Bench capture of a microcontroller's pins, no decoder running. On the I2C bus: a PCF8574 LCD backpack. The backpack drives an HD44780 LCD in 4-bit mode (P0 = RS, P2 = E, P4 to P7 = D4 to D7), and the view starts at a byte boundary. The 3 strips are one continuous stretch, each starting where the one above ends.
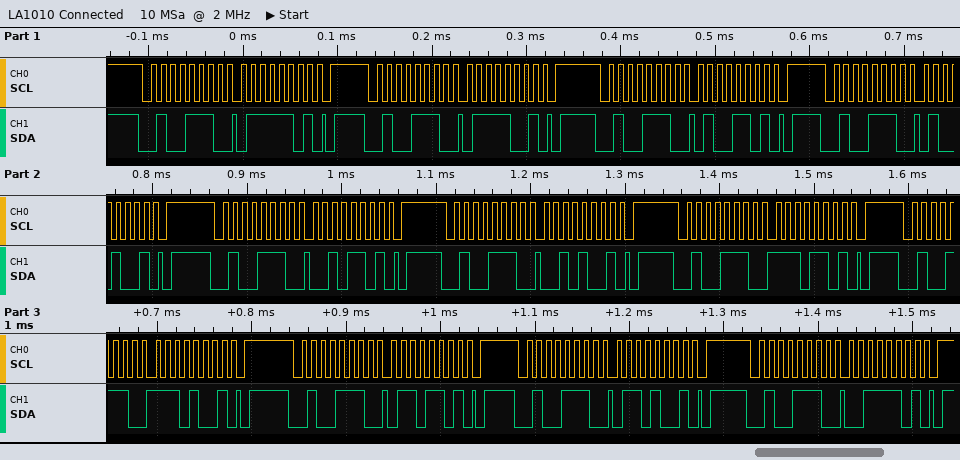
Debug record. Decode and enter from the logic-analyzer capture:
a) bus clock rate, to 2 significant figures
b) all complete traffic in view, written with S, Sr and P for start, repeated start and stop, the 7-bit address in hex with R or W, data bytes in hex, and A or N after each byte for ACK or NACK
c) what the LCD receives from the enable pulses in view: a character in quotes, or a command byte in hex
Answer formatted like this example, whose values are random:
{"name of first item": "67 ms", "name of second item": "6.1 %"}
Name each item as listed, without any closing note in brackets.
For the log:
{"bus clock rate, to 2 significant figures": "100 kHz", "all complete traffic in view, written with S, Sr and P for start, repeated start and stop, the 7-bit address in hex with R or W, data bytes in hex, and A or N after each byte for ACK or NACK": "S 27W A 7D A P S 27W A 79 A P S 27W A 4D A P S 27W A 49 A P S 27W A 2D A P S 27W A 29 A P S 27W A ED A P S 27W A E9 A P S 27W A 6D A P S 27W A 69 A P S 27W A 3D A P", "what the LCD receives from the enable pulses in view: a character in quotes, or a command byte in hex": "'t' '.'"}
